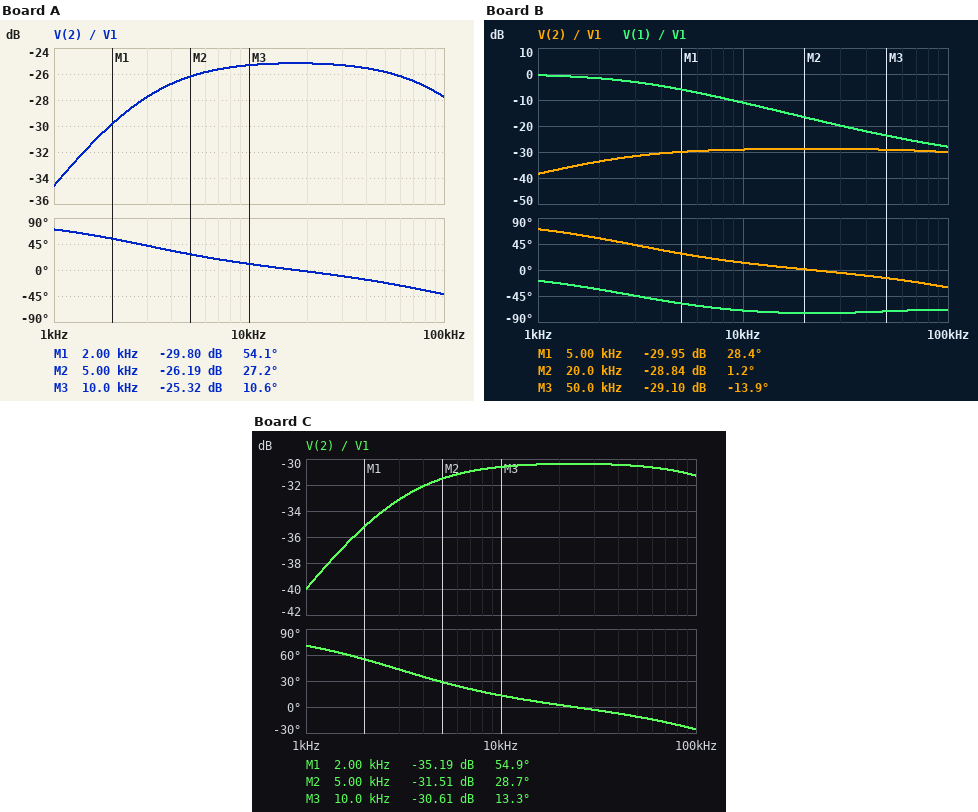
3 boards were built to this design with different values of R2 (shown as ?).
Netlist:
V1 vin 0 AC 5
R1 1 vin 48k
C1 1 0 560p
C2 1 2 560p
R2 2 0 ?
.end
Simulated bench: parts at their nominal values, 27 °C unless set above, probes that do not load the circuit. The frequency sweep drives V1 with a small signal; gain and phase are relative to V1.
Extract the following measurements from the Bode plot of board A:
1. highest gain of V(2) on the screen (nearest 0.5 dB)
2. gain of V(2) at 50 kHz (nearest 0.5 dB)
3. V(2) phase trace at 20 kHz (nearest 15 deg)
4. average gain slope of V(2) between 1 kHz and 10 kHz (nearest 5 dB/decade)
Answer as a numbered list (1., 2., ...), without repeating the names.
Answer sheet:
1. -25.0 dB
2. -26.0 dB
3. 0 deg
4. 10 dB/decade
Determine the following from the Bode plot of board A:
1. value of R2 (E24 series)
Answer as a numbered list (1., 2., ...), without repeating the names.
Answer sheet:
1. 5.6 kΩ
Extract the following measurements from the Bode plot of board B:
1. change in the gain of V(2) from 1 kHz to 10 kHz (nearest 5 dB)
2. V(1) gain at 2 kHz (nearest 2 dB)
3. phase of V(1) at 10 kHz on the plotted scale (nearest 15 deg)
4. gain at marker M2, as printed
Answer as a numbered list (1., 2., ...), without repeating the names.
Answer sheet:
1. 10 dB
2. -2 dB
3. -75 deg
4. -28.84 dB
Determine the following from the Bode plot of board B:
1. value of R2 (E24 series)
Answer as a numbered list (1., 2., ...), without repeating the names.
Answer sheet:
1. 3.6 kΩ
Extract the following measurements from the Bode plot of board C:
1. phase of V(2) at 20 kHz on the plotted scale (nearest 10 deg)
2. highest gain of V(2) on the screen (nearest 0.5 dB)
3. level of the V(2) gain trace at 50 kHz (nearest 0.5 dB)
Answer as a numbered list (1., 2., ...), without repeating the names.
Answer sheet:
1. 0 deg
2. -30.5 dB
3. -30.5 dB
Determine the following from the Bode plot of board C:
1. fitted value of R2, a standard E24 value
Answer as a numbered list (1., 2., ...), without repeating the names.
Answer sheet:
1. 3 kΩ
